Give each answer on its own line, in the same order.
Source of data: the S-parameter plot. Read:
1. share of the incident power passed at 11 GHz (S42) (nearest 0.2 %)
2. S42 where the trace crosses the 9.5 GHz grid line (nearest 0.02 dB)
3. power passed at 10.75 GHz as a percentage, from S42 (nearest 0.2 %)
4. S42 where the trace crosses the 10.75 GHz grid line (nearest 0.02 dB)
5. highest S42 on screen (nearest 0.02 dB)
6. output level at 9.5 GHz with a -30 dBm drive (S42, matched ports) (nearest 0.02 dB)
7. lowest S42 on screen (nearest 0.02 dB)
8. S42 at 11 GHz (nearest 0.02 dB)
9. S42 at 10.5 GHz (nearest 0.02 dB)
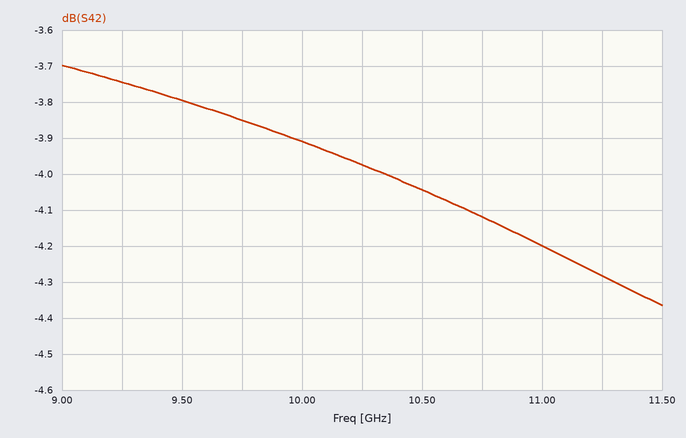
38.0 %
-3.80 dB
38.8 %
-4.12 dB
-3.70 dB
-33.80 dBm
-4.36 dB
-4.20 dB
-4.04 dB
